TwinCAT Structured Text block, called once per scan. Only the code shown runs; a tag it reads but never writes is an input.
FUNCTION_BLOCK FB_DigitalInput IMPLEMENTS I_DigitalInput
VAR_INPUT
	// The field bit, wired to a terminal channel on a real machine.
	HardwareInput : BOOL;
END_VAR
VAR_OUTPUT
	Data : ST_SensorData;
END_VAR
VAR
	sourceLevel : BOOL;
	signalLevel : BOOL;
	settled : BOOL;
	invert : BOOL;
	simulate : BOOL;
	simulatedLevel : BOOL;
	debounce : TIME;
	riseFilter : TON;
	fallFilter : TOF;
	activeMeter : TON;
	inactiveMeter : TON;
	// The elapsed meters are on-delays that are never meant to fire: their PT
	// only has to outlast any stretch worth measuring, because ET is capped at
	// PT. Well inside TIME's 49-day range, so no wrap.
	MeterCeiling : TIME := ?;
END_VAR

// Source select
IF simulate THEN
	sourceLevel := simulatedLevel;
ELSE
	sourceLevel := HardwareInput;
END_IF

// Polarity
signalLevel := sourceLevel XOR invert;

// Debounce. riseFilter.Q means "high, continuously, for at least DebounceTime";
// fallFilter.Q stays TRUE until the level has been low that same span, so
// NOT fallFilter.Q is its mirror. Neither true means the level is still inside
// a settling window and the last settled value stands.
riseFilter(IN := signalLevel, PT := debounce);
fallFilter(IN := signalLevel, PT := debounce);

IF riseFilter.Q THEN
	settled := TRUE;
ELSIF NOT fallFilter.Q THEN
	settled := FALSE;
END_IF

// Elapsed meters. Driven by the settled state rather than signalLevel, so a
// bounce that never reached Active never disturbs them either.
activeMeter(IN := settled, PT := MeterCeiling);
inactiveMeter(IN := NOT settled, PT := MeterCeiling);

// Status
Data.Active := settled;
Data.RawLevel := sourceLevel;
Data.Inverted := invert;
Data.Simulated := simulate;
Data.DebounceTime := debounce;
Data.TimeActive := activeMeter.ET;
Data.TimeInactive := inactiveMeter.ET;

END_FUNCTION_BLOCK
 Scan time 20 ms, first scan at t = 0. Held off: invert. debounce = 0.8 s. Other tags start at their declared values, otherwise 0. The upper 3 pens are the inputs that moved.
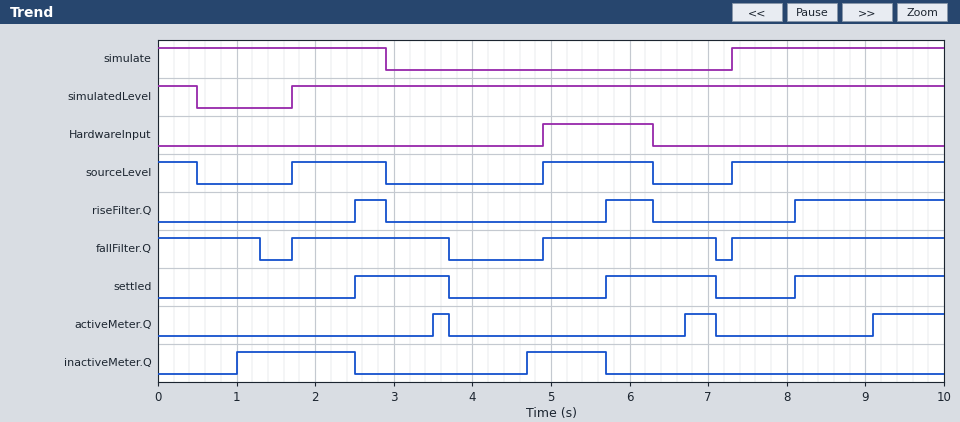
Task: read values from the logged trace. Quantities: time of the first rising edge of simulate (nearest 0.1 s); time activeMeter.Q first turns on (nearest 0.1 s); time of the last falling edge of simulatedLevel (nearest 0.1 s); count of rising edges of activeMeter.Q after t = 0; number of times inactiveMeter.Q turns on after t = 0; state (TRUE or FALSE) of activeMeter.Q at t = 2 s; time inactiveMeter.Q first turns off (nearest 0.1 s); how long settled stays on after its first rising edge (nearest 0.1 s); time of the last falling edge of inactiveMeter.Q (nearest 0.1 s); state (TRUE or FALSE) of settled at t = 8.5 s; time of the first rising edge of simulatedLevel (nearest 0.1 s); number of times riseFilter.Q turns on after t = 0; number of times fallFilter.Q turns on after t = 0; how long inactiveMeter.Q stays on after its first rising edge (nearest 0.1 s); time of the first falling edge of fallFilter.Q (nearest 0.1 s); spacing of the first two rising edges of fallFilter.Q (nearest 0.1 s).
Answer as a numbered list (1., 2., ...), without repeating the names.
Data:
1. 7.3 s
2. 3.5 s
3. 0.5 s
4. 3
5. 2
6. FALSE
7. 2.5 s
8. 1.2 s
9. 5.7 s
10. TRUE
11. 1.7 s
12. 3
13. 3
14. 1.5 s
15. 1.3 s
16. 3.2 s
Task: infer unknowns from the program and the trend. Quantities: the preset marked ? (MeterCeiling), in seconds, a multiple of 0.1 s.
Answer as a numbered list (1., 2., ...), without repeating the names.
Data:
1. 1.0 s
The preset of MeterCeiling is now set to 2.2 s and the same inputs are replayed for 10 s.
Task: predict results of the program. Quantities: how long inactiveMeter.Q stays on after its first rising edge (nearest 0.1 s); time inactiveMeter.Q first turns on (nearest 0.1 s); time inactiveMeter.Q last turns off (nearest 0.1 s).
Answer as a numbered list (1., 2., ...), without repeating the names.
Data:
1. 0.3 s
2. 2.2 s
3. 2.5 s
